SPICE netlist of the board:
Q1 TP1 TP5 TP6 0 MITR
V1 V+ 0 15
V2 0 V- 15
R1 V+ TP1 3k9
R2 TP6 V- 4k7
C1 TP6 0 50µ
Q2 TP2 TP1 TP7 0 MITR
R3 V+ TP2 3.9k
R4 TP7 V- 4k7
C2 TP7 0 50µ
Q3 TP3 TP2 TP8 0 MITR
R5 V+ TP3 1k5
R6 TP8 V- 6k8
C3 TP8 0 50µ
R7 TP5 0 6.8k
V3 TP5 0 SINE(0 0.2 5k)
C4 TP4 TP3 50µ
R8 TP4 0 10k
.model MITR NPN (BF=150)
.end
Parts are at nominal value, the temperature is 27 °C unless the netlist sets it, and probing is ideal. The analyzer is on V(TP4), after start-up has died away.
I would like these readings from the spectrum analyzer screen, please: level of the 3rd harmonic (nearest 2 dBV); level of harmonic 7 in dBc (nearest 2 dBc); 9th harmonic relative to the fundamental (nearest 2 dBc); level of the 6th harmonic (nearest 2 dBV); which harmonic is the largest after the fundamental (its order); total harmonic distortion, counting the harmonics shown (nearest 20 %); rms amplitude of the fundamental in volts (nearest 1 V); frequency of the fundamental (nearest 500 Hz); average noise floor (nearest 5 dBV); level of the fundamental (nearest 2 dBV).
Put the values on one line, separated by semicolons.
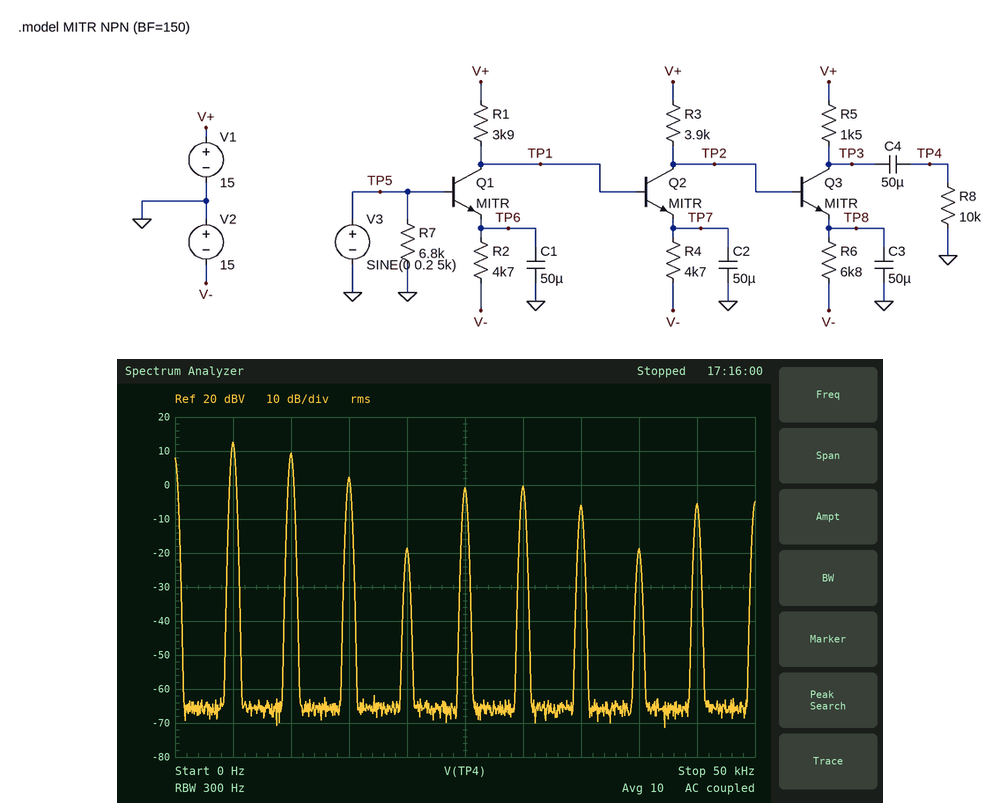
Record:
2 dBV; -18 dBc; -18 dBc; 0 dBV; 2; 80 %; 4 V; 5.0 kHz; -65 dBV; 12 dBV
